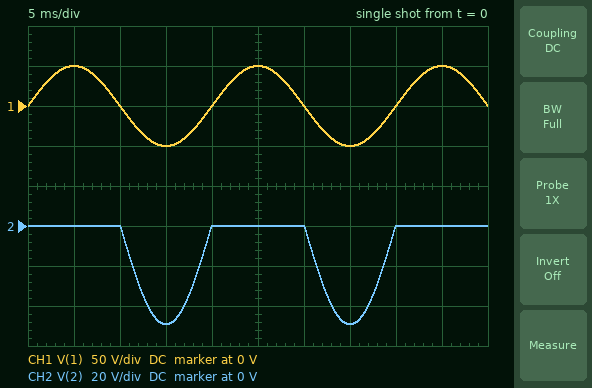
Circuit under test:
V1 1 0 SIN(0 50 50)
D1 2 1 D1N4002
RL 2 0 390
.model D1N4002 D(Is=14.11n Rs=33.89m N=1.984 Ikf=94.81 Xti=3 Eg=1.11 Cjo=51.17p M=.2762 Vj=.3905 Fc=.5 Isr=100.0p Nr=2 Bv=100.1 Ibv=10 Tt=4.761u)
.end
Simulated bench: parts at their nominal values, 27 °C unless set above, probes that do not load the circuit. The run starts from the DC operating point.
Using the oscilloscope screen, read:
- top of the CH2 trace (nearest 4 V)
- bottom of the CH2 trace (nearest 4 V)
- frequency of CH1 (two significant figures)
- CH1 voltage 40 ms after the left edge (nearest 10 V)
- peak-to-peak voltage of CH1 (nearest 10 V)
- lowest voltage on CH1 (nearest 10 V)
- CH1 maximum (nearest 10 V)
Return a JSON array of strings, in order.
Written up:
["0 V", "-48 V", "50 Hz", "0 V", "100 V", "-50 V", "50 V"]
